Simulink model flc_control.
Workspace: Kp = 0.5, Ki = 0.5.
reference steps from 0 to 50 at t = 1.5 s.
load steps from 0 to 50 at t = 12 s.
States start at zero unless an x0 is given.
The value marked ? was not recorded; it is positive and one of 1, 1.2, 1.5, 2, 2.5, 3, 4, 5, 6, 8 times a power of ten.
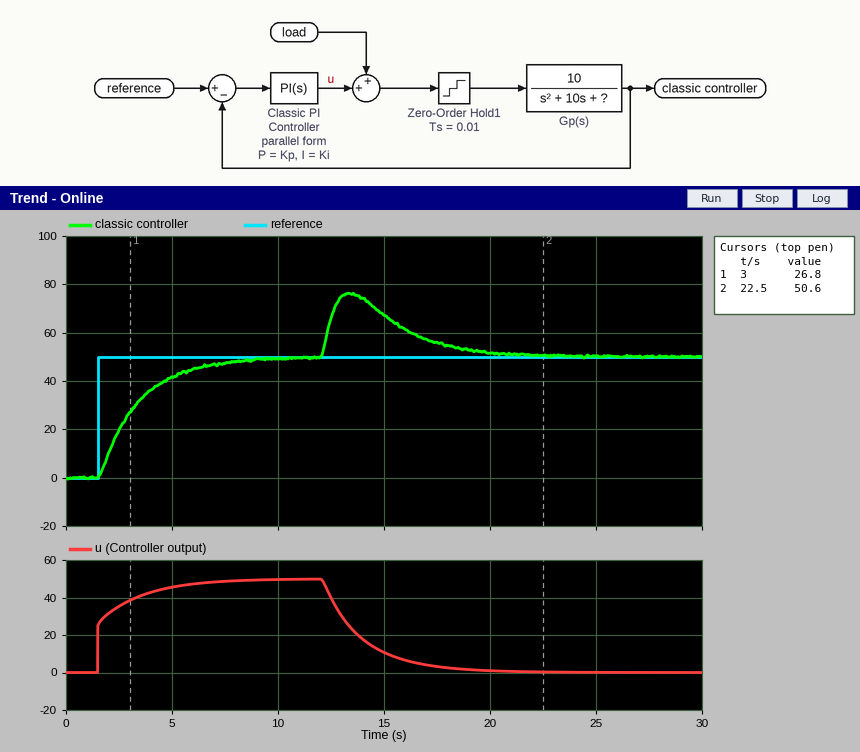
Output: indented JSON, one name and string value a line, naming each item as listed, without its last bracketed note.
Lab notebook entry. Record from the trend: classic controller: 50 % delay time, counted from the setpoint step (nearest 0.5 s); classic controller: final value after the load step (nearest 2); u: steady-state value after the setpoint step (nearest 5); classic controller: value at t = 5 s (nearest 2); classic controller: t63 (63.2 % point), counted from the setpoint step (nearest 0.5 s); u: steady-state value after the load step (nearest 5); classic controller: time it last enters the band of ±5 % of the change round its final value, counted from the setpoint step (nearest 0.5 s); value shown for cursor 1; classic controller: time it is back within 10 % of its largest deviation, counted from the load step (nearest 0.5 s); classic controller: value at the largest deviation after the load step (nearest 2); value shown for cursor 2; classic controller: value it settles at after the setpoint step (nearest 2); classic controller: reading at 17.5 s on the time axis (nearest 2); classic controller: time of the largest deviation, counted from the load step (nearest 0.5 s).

{
  "classic controller: 50 % delay time, counted from the setpoint step": "1.5 s",
  "classic controller: final value after the load step": "50",
  "u: steady-state value after the setpoint step": "50",
  "classic controller: value at t = 5 s": "42",
  "classic controller: t63 (63.2 % point), counted from the setpoint step": "2.0 s",
  "u: steady-state value after the load step": "0",
  "classic controller: time it last enters the band of ±5 % of the change round its final value, counted from the setpoint step": "6.0 s",
  "value shown for cursor 1": "26.8",
  "classic controller: time it is back within 10 % of its largest deviation, counted from the load step": "7.0 s",
  "classic controller: value at the largest deviation after the load step": "76",
  "value shown for cursor 2": "50.6",
  "classic controller: value it settles at after the setpoint step": "50",
  "classic controller: reading at 17.5 s on the time axis": "56",
  "classic controller: time of the largest deviation, counted from the load step": "1.5 s"
}
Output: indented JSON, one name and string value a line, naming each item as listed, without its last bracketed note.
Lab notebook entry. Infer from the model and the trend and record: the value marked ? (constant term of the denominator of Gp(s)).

{
  "the value marked ? (constant term of the denominator of Gp(s))": "10"
}
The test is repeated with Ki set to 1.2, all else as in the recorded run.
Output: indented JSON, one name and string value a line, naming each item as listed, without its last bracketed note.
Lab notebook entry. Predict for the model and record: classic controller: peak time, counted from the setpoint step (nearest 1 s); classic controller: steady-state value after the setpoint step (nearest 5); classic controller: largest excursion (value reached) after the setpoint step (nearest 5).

{
  "classic controller: peak time, counted from the setpoint step": "3 s",
  "classic controller: steady-state value after the setpoint step": "50",
  "classic controller: largest excursion (value reached) after the setpoint step": "55"
}
